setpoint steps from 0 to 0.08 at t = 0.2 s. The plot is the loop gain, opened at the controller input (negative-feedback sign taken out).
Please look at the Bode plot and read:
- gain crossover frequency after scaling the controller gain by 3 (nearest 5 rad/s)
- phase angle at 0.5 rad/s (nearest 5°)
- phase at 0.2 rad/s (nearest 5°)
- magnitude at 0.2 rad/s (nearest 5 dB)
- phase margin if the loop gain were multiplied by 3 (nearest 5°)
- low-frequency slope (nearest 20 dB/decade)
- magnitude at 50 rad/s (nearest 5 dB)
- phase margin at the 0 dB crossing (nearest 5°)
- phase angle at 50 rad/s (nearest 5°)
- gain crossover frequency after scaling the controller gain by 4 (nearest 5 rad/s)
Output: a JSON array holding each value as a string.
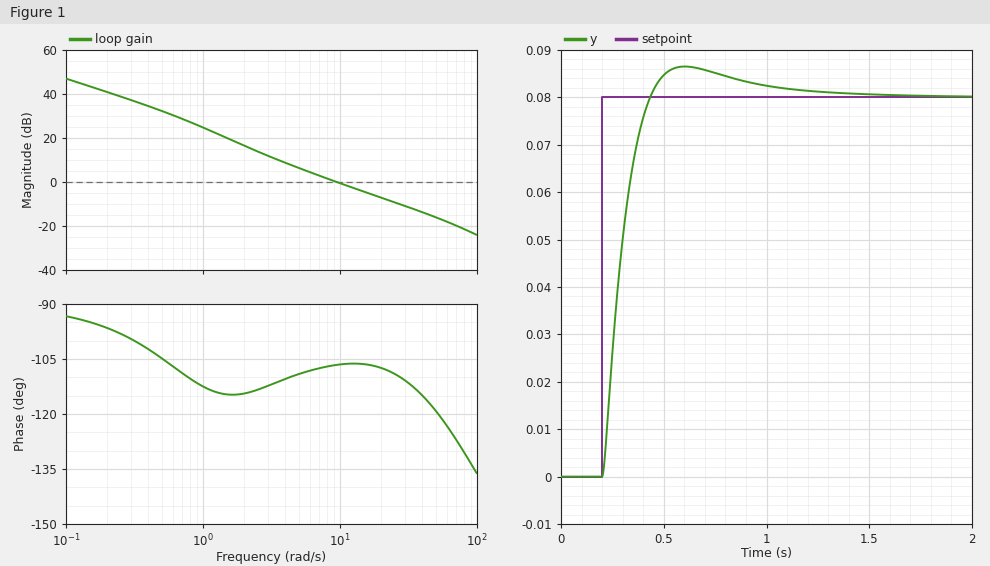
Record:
["25 rad/s", "-105°", "-95°", "40 dB", "70°", "-20 dB/decade", "-15 dB", "75°", "-120°", "35 rad/s"]
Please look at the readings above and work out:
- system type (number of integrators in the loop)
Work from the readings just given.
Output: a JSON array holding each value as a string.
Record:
["1"]
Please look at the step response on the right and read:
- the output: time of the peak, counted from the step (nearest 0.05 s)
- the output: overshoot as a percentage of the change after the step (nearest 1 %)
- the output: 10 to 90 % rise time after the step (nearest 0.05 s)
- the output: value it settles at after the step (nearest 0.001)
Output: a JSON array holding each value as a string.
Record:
["0.40 s", "8 %", "0.15 s", "0.080"]
